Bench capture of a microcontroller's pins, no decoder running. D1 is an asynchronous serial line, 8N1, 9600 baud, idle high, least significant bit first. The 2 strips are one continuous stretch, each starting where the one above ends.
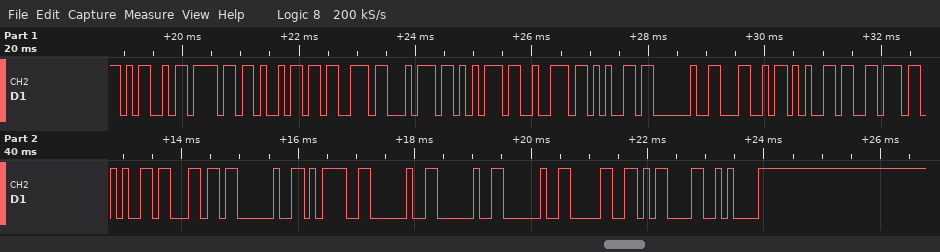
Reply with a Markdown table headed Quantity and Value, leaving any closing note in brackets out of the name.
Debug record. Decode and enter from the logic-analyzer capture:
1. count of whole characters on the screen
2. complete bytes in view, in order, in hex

| Quantity | Value |
|---|---|
| count of whole characters on the screen | 22 |
| complete bytes in view, in order, in hex | 4D 6F 69 73 74 75 72 65 20 4C 65 76 65 6C 20 3D 20 20 20 30 0D 0A |
